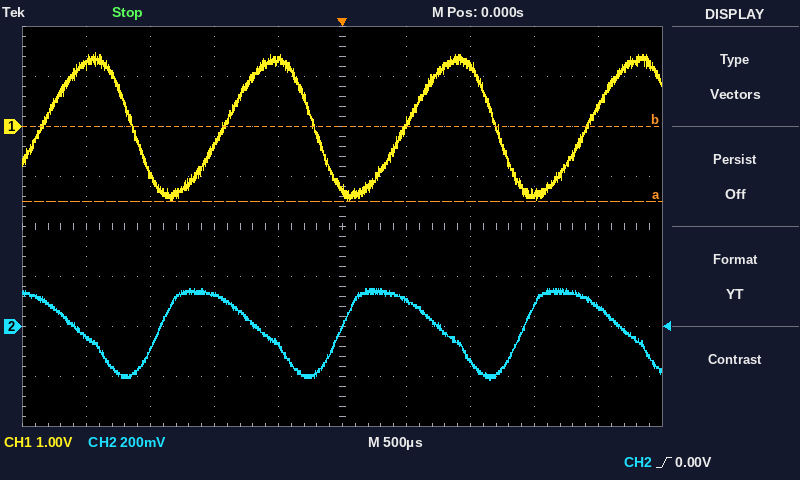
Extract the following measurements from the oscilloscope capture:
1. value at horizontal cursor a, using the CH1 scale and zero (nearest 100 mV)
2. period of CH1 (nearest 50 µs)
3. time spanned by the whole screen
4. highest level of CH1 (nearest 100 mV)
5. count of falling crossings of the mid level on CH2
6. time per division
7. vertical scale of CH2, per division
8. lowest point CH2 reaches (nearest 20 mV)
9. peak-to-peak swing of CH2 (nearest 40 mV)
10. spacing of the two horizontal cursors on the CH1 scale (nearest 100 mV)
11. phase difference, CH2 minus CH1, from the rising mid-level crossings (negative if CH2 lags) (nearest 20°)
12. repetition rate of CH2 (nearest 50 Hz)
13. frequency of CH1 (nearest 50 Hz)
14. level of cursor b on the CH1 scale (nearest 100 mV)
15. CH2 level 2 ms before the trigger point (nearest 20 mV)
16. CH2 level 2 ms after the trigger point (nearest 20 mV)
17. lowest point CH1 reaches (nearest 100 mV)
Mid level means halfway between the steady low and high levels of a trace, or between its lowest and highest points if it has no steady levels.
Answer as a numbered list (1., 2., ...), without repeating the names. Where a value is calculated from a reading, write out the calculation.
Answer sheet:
1. -1.5 V
2. 1.40 ms
3. 5 ms
4. 1.5 V
5. 4
6. 500 µs
7. 200 mV
8. -220 mV
9. 360 mV
10. 1.5 V
11. +140°
12. 700 Hz
13. 1 / 1.40 ms ≈ 714 Hz, so 700 Hz to the nearest 50 Hz
14. 0.0 V
15. -40 mV
16. 80 mV
17. -1.5 V
